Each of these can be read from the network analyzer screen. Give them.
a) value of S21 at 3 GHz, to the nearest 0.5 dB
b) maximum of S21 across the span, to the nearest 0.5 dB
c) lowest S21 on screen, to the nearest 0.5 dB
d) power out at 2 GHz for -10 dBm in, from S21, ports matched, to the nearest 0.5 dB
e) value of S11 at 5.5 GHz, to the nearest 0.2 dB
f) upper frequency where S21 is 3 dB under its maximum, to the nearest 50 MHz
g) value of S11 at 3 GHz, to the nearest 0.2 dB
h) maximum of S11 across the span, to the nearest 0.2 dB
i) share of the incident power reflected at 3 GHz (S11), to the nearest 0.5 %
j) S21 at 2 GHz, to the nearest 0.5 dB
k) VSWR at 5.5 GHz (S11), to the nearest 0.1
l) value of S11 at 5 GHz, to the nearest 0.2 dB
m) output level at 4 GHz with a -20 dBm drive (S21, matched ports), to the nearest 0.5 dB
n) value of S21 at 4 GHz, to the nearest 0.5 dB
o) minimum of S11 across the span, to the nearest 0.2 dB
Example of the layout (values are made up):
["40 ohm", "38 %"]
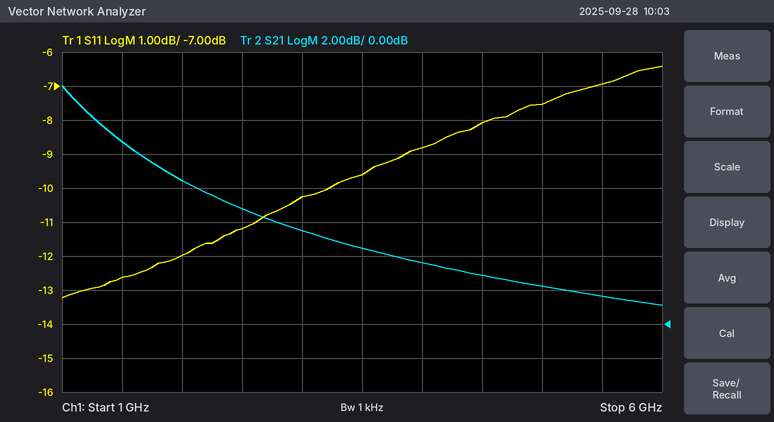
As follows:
["5.5 dB", "14.0 dB", "1.0 dB", "-1.5 dBm", "-7.0 dB", "1.45 GHz", "-10.2 dB", "-6.4 dB", "9.5 %", "8.5 dB", "2.6", "-7.6 dB", "-16.5 dBm", "3.5 dB", "-13.2 dB"]
